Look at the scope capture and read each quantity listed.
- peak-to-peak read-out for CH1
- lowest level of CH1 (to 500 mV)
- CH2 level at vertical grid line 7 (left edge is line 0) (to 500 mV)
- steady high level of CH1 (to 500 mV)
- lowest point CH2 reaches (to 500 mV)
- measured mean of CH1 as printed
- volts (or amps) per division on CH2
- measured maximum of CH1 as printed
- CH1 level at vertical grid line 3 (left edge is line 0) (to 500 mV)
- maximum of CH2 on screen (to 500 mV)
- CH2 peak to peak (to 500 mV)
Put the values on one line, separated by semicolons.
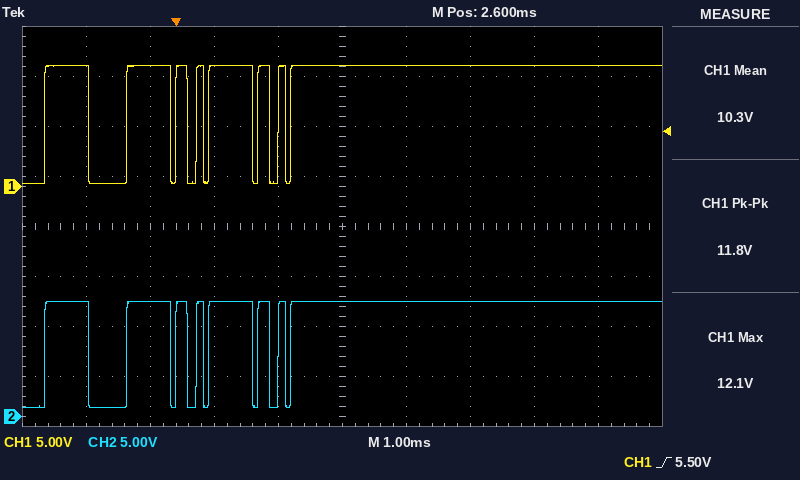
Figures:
11.8 V; 500 mV; 11.5 V; 12.0 V; 1.0 V; 10.3 V; 5 V; 12.1 V; 12.0 V; 11.5 V; 10.5 V
